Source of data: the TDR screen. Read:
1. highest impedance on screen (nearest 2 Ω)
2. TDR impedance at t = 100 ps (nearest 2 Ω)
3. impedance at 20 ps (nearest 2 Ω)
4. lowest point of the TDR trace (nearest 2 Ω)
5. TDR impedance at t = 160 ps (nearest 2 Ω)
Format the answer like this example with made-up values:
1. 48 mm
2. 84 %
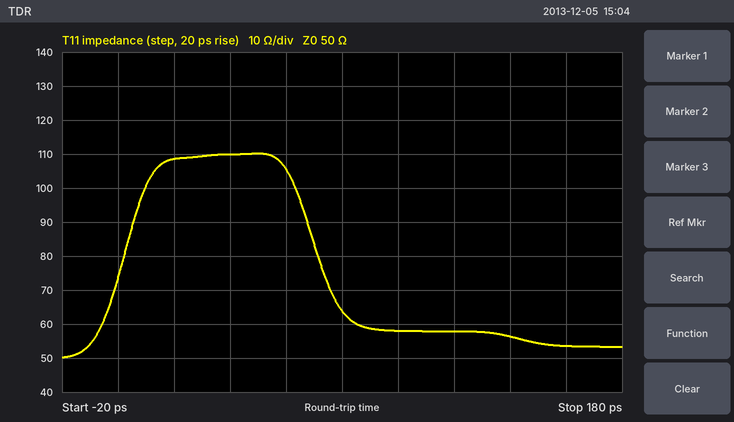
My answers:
1. 110 Ω
2. 58 Ω
3. 108 Ω
4. 50 Ω
5. 54 Ω
